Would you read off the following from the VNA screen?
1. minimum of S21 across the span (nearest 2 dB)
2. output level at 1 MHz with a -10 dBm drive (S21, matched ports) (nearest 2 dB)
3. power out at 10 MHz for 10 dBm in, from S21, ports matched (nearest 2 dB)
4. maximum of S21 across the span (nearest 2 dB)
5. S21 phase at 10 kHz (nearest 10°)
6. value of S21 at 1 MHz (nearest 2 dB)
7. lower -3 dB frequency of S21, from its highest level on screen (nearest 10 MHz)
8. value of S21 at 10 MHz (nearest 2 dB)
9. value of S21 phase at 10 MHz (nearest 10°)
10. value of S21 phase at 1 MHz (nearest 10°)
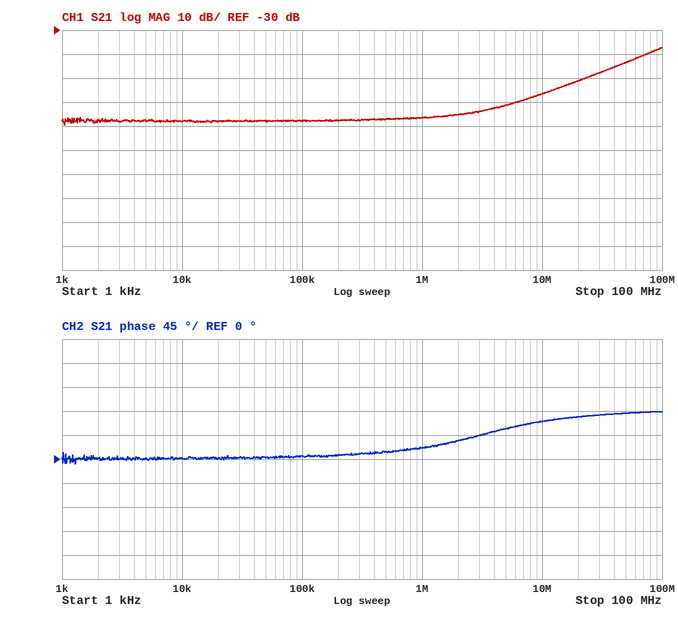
-70 dB
-76 dBm
-46 dBm
-38 dB
0°
-66 dB
70 MHz
-56 dB
70°
20°
